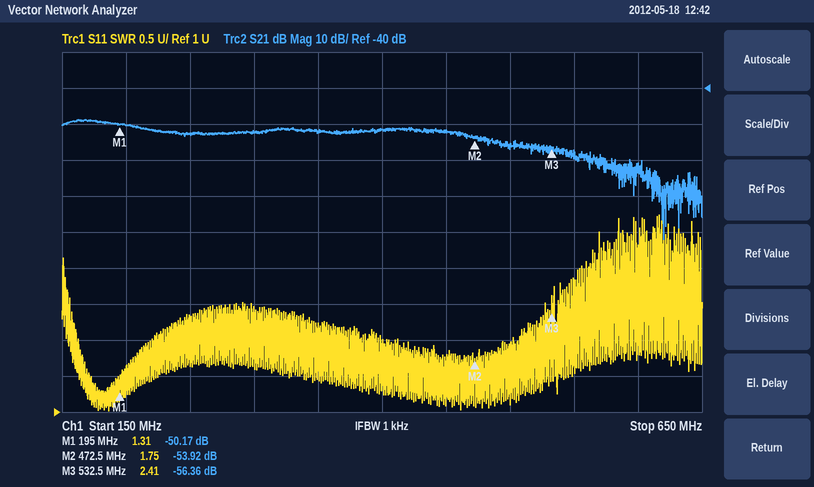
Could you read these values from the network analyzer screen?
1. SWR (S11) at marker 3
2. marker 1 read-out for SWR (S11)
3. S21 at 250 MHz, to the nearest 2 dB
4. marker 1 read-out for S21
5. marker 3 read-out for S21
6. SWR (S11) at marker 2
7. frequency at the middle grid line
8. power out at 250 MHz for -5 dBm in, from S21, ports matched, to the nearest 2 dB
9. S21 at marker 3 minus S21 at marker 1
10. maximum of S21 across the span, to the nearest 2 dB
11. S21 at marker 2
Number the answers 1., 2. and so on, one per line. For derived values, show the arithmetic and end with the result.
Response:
1. 2.41
2. 1.31
3. -52 dB
4. -50.17 dB
5. -56.36 dB
6. 1.75
7. 400 MHz
8. -5 dBm + (-52 dB) = -58 dBm
9. -56.36 − (-50.17) = -6.19 dB
10. -48 dB
11. -53.92 dB
